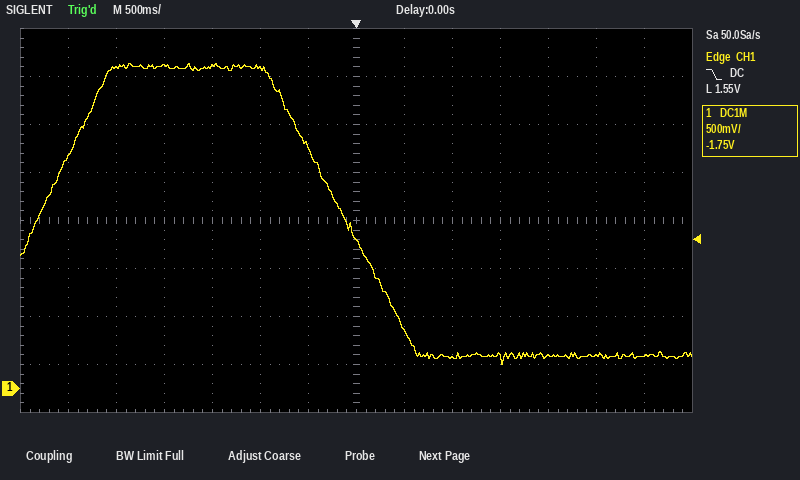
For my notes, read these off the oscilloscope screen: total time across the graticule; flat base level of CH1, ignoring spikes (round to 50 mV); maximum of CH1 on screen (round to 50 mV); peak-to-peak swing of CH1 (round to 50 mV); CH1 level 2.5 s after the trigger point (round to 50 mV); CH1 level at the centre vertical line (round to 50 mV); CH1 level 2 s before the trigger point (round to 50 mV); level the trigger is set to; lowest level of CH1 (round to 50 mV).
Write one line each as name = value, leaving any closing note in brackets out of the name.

total time across the graticule = 7 s
flat base level of CH1, ignoring spikes = 350 mV
maximum of CH1 on screen = 3.40 V
peak-to-peak swing of CH1 = 3.15 V
CH1 level 2.5 s after the trigger point = 350 mV
CH1 level at the centre vertical line = 1.55 V
CH1 level 2 s before the trigger point = 3.35 V
level the trigger is set to = 1.55 V
lowest level of CH1 = 250 mV
